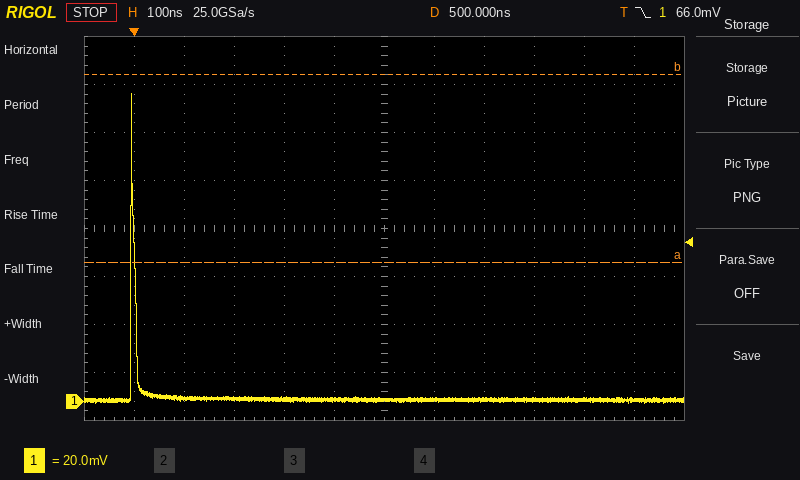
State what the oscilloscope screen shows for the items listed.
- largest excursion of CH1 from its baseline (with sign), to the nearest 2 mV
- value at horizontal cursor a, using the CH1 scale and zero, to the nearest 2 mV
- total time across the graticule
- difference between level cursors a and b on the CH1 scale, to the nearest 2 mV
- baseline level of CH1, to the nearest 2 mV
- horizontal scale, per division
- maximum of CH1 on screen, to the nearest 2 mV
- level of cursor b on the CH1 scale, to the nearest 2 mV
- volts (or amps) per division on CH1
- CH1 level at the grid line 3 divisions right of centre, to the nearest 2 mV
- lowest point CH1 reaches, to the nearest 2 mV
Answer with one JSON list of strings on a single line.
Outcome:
["+128 mV", "58 mV", "1.2 µs", "78 mV", "0 mV", "100 ns", "128 mV", "136 mV", "20 mV", "0 mV", "0 mV"]
